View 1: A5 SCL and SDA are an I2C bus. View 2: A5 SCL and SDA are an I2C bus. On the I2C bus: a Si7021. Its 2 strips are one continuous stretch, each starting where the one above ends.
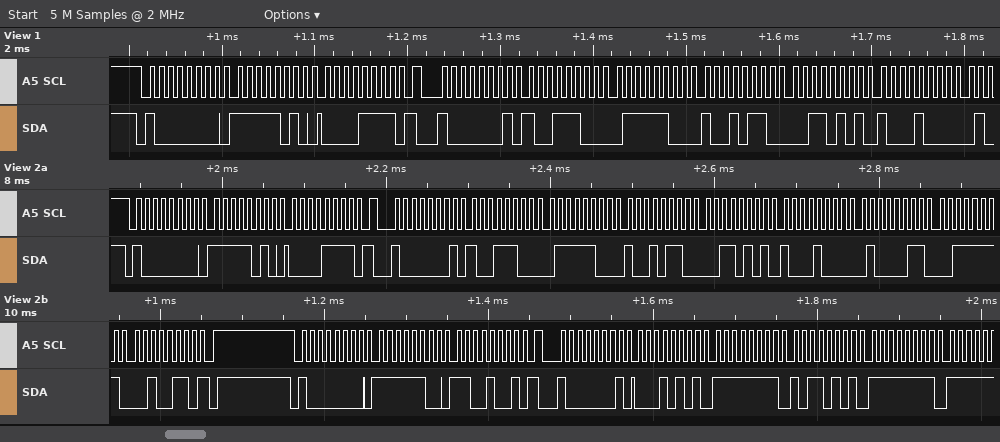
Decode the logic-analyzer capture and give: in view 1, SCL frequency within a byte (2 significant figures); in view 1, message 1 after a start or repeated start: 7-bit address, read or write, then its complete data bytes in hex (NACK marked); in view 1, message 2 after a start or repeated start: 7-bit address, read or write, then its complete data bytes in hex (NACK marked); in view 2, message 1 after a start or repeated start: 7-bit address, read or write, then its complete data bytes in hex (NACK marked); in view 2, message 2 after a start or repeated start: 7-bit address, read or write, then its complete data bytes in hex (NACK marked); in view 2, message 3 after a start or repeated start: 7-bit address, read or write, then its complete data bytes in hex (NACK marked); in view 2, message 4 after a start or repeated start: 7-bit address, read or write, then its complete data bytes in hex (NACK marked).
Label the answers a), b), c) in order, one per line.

a) 100 kHz
b) 0x40 write: FA 0F
c) 0x40 read: 9C 7C 96 35 88
d) 0x40 write: FA 0F
e) 0x40 read: 9C 7C 96 35 88 43 3F 26 NACK
f) 0x40 write: FC C9
g) 0x40 read: 15 FF B5 FF
